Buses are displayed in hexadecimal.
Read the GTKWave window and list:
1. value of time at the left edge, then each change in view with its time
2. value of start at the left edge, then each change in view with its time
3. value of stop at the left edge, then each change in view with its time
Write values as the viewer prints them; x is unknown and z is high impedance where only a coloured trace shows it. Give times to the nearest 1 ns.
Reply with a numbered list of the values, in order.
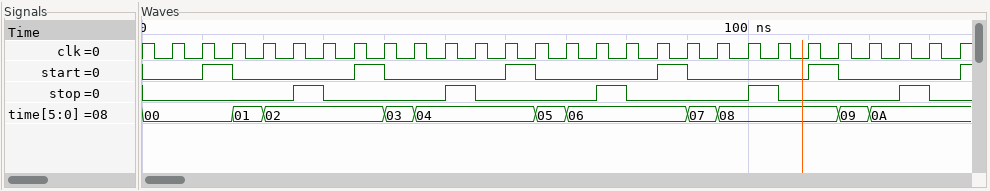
1. 00, 01 at 15 ns, 02 at 20 ns, 03 at 40 ns, 04 at 45 ns, 05 at 65 ns, 06 at 70 ns, 07 at 90 ns, 08 at 95 ns, 09 at 115 ns, 0A at 120 ns
2. 0, 1 at 10 ns, 0 at 15 ns, 1 at 35 ns, 0 at 40 ns, 1 at 60 ns, 0 at 65 ns, 1 at 85 ns, 0 at 90 ns, 1 at 110 ns, 0 at 115 ns, 1 at 135 ns
3. 0, 1 at 25 ns, 0 at 30 ns, 1 at 50 ns, 0 at 55 ns, 1 at 75 ns, 0 at 80 ns, 1 at 100 ns, 0 at 105 ns, 1 at 125 ns, 0 at 130 ns
